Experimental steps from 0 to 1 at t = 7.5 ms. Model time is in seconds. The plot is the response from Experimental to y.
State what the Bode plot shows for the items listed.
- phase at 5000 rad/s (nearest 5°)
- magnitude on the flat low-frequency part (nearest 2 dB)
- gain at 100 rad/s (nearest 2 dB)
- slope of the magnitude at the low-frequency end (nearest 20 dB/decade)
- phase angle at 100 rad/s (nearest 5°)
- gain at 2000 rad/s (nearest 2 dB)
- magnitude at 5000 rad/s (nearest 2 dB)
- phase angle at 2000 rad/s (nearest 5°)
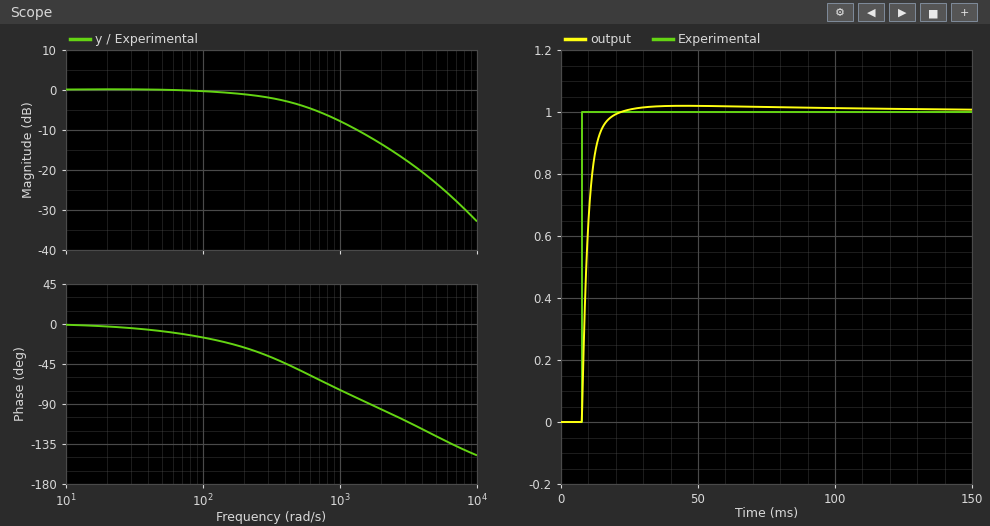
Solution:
-125°
0 dB
0 dB
0 dB/decade
-15°
-14 dB
-24 dB
-95°
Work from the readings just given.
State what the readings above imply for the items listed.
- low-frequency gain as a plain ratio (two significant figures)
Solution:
1.0
